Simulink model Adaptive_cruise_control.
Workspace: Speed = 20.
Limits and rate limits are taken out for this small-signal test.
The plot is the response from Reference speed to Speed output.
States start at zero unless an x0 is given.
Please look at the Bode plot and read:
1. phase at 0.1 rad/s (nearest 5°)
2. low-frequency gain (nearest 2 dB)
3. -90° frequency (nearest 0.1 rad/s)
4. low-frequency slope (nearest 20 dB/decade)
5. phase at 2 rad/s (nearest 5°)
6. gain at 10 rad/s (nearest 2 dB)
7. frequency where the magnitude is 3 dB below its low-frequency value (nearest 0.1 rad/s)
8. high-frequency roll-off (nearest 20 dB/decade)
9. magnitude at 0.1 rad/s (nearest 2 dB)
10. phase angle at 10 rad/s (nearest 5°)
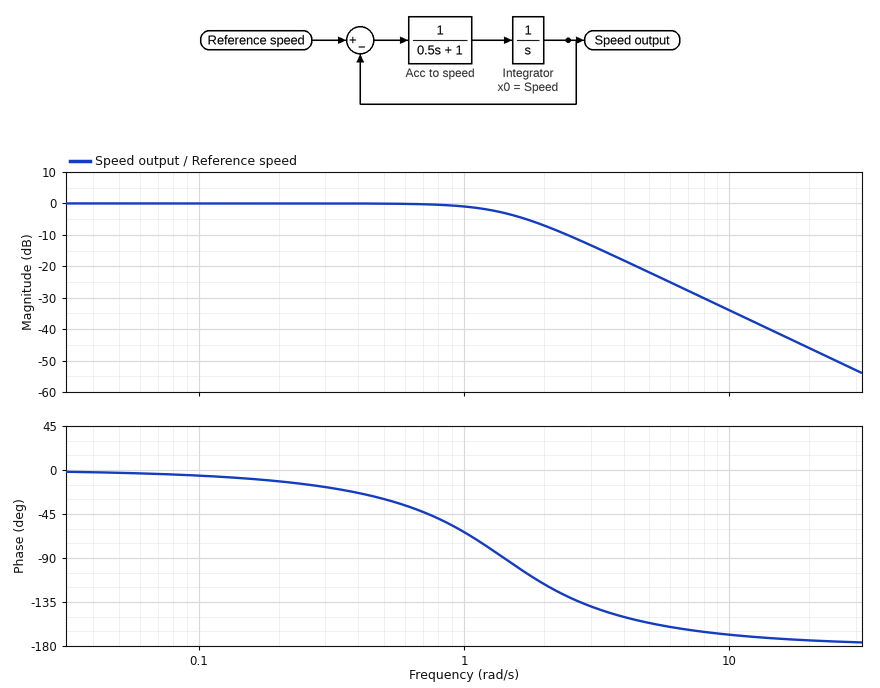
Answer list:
-5°
0 dB
1.4 rad/s
0 dB/decade
-115°
-34 dB
1.4 rad/s
-40 dB/decade
0 dB
-170°
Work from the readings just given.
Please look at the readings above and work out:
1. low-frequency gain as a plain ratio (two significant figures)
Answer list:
1.0
